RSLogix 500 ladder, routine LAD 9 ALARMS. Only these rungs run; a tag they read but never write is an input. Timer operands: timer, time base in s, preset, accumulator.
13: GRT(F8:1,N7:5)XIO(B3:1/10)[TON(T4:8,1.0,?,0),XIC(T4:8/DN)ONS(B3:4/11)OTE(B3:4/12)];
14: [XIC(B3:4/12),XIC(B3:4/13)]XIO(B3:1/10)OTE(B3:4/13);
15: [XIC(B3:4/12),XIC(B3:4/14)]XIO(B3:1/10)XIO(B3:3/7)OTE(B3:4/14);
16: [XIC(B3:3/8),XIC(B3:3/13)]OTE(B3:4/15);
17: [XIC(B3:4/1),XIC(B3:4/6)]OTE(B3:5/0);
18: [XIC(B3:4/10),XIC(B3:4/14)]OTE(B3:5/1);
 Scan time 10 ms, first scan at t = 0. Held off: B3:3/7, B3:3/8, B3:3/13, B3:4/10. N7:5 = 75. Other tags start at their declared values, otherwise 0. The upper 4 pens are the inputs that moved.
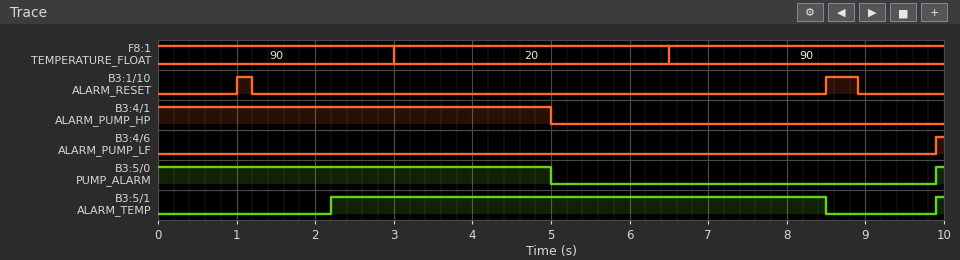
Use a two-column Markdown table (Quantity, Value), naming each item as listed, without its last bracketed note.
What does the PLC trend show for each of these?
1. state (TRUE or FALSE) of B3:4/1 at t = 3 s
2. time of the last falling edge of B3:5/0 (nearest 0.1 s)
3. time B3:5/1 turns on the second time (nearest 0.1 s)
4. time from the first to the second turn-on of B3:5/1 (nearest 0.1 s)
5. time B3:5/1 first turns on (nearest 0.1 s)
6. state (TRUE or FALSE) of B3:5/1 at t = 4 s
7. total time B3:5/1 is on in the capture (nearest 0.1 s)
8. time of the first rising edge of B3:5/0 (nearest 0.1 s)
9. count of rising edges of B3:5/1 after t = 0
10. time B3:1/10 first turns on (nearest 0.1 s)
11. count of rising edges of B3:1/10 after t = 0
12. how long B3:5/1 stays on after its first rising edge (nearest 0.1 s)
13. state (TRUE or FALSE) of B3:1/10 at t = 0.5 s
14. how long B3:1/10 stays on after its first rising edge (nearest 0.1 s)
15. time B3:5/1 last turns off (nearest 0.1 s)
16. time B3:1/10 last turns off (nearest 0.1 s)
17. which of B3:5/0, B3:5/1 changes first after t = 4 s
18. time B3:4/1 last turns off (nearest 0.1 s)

| Quantity | Value |
|---|---|
| state (TRUE or FALSE) of B3:4/1 at t = 3 s | TRUE |
| time of the last falling edge of B3:5/0 | 5.0 s |
| time B3:5/1 turns on the second time | 9.9 s |
| time from the first to the second turn-on of B3:5/1 | 7.7 s |
| time B3:5/1 first turns on | 2.2 s |
| state (TRUE or FALSE) of B3:5/1 at t = 4 s | TRUE |
| total time B3:5/1 is on in the capture | 6.4 s |
| time of the first rising edge of B3:5/0 | 9.9 s |
| count of rising edges of B3:5/1 after t = 0 | 2 |
| time B3:1/10 first turns on | 1.0 s |
| count of rising edges of B3:1/10 after t = 0 | 2 |
| how long B3:5/1 stays on after its first rising edge | 6.3 s |
| state (TRUE or FALSE) of B3:1/10 at t = 0.5 s | FALSE |
| how long B3:1/10 stays on after its first rising edge | 0.2 s |
| time B3:5/1 last turns off | 8.5 s |
| time B3:1/10 last turns off | 8.9 s |
| which of B3:5/0, B3:5/1 changes first after t = 4 s | B3:5/0 |
| time B3:4/1 last turns off | 5.0 s |
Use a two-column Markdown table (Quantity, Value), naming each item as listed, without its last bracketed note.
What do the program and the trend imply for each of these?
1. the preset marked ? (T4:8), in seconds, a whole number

| Quantity | Value |
|---|---|
| the preset marked ? (T4:8), in seconds, a whole number | 1 s |
